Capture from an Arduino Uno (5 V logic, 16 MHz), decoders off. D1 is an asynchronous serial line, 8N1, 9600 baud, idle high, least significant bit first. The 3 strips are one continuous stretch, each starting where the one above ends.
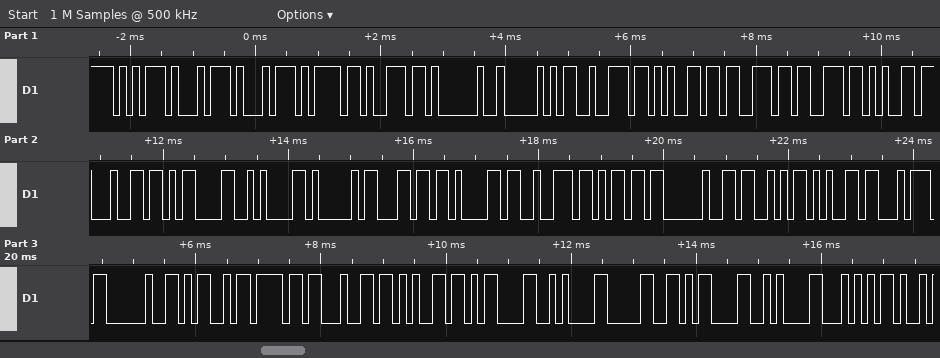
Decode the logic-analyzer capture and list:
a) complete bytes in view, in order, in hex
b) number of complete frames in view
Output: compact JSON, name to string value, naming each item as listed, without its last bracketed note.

{"complete bytes in view, in order, in hex": "0x75 0x74 0x74 0x6F 0x6E 0x20 0x50 0x72 0x65 0x73 0x73 0x65 0x64 0x0D 0x0A 0x41 0x6C 0x61 0x72 0x6D 0x20 0x53 0x65 0x74 0x20 0x4D 0x6F 0x64 0x65 0x0D 0x0A 0x30 0x0D 0x0A 0x54", "number of complete frames in view": "35"}
